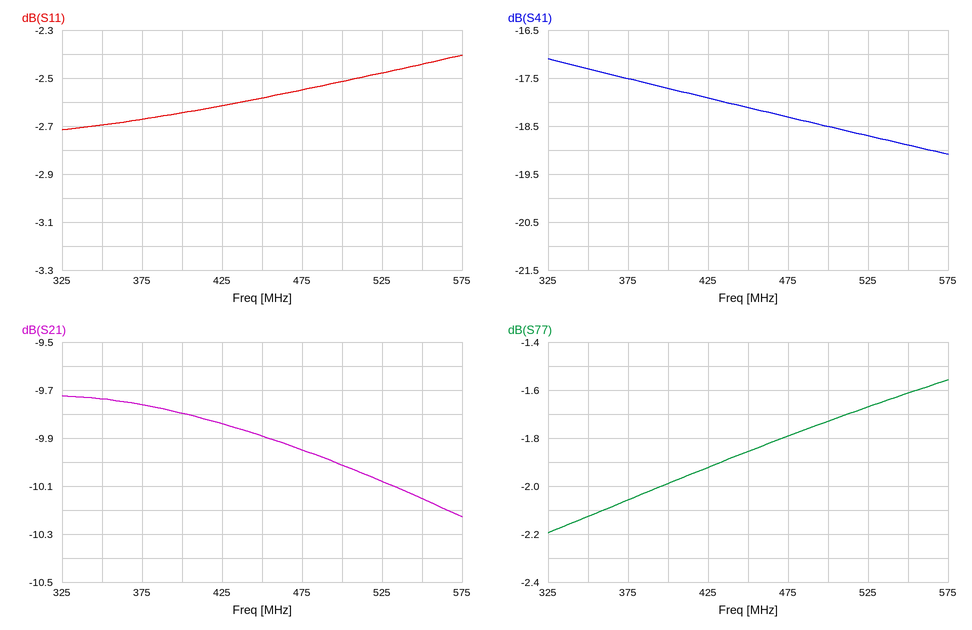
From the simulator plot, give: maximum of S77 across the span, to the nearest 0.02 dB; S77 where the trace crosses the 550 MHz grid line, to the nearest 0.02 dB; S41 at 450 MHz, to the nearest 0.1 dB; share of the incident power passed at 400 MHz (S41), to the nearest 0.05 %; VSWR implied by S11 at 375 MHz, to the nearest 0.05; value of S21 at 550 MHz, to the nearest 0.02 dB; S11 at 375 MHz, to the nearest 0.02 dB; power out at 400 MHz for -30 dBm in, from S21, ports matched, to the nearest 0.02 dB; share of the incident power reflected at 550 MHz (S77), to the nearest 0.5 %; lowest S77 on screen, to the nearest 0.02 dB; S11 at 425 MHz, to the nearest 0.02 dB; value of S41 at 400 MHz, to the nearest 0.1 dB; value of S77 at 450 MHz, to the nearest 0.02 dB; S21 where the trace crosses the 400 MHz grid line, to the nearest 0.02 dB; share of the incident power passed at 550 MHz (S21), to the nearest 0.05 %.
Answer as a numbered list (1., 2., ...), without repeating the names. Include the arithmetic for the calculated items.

1. -1.56 dB
2. -1.62 dB
3. -18.1 dB
4. 10^(-17.7/10) ≈ 1.70 %
5. |Γ| = 10^(-2.68/20) = 0.7345; VSWR = (1 + 0.7345)/(1 − 0.7345) ≈ 6.53, so 6.55 to the nearest 0.05
6. -10.16 dB
7. -2.68 dB
8. -30 dBm + (-9.80 dB) = -39.80 dBm
9. 10^(-1.62/10) ≈ 68.9 %, so 69.0 % to the nearest 0.5 %
10. -2.20 dB
11. -2.62 dB
12. -17.7 dB
13. -1.86 dB
14. -9.80 dB
15. 10^(-10.16/10) ≈ 9.64 %, so 9.65 % to the nearest 0.05 %
